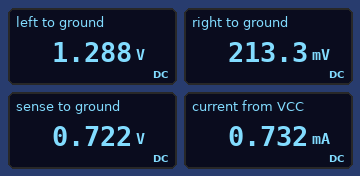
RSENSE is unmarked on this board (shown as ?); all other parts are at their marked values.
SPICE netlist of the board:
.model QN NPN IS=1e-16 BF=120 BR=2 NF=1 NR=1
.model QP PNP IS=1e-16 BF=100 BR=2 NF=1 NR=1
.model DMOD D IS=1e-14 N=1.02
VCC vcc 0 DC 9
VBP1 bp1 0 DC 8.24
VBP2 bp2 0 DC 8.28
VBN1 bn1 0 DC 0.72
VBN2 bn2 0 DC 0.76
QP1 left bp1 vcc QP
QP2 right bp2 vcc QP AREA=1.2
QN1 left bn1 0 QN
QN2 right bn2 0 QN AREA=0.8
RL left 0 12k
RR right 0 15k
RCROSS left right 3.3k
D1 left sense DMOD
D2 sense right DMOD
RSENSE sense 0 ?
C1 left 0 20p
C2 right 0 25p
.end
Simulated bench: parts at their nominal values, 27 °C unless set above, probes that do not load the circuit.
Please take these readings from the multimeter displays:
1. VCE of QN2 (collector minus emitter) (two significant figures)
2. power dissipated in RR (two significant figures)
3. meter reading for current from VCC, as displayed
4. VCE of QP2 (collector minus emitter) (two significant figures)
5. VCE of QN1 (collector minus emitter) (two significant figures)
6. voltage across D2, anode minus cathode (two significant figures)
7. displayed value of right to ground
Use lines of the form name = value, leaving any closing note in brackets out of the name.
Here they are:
VCE of QN2 (collector minus emitter) = 210 mV
power dissipated in RR = 3.0 µW
meter reading for current from VCC, as displayed = 0.732 mA
VCE of QP2 (collector minus emitter) = -8.8 V
VCE of QN1 (collector minus emitter) = 1.3 V
voltage across D2, anode minus cathode = 510 mV
displayed value of right to ground = 213.3 mV
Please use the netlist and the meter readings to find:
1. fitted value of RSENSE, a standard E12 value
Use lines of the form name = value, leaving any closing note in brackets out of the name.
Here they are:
fitted value of RSENSE, a standard E12 value = 39 kΩ
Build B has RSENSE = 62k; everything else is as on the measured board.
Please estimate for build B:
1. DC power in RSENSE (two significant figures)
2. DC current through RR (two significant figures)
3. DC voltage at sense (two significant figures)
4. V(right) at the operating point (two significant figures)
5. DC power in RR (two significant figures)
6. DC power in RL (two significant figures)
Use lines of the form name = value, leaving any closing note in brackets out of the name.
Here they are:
DC power in RSENSE = 9.6 µW
DC current through RR = 17 µA
DC voltage at sense = 770 mV
V(right) at the operating point = 250 mV
DC power in RR = 4.2 µW
DC power in RL = 150 µW
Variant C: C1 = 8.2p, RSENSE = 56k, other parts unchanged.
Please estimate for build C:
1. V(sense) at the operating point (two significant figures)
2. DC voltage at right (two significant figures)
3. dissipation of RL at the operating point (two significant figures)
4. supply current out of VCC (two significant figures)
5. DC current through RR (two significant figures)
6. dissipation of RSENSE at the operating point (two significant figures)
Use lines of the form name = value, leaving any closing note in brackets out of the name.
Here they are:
V(sense) at the operating point = 760 mV
DC voltage at right = 240 mV
dissipation of RL at the operating point = 150 µW
supply current out of VCC = 730 µA
DC current through RR = 16 µA
dissipation of RSENSE at the operating point = 10 µW
